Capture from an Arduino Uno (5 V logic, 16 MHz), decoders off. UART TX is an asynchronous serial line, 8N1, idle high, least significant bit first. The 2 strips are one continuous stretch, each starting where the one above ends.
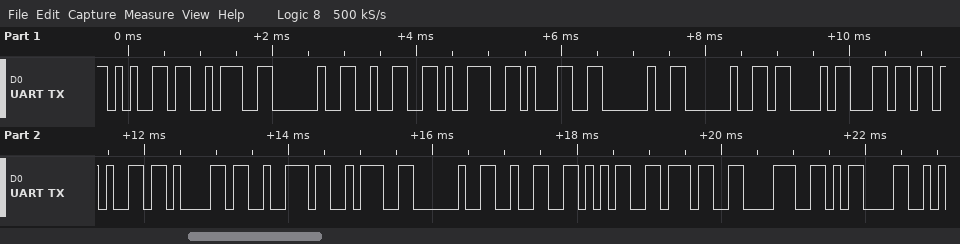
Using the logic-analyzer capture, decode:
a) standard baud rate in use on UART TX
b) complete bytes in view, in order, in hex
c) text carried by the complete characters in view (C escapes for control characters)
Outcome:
9600 baud
65 3A 20 32 39 31 20 20 43 6C 65 61 72 3A 20 32 35 37 38 0D
"e: 291  Clear: 2578\r"
